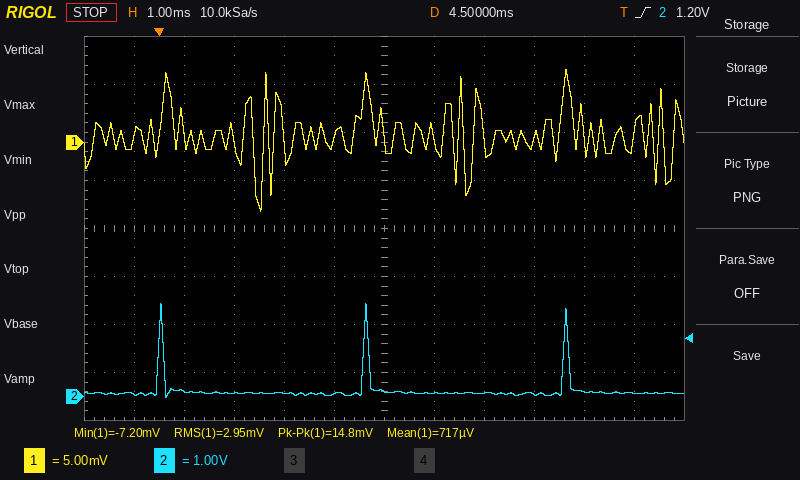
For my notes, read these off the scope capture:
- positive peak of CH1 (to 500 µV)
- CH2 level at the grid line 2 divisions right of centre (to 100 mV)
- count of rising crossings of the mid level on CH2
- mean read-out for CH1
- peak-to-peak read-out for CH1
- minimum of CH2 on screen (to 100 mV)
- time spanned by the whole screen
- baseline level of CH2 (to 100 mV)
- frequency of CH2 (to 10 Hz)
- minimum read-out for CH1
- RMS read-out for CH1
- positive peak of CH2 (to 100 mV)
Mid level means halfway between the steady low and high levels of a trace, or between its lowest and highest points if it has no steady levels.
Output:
7.5 mV
100 mV
3
717 µV
14.8 mV
0.0 V
12 ms
100 mV
250 Hz
-7.20 mV
2.95 mV
1.9 V
